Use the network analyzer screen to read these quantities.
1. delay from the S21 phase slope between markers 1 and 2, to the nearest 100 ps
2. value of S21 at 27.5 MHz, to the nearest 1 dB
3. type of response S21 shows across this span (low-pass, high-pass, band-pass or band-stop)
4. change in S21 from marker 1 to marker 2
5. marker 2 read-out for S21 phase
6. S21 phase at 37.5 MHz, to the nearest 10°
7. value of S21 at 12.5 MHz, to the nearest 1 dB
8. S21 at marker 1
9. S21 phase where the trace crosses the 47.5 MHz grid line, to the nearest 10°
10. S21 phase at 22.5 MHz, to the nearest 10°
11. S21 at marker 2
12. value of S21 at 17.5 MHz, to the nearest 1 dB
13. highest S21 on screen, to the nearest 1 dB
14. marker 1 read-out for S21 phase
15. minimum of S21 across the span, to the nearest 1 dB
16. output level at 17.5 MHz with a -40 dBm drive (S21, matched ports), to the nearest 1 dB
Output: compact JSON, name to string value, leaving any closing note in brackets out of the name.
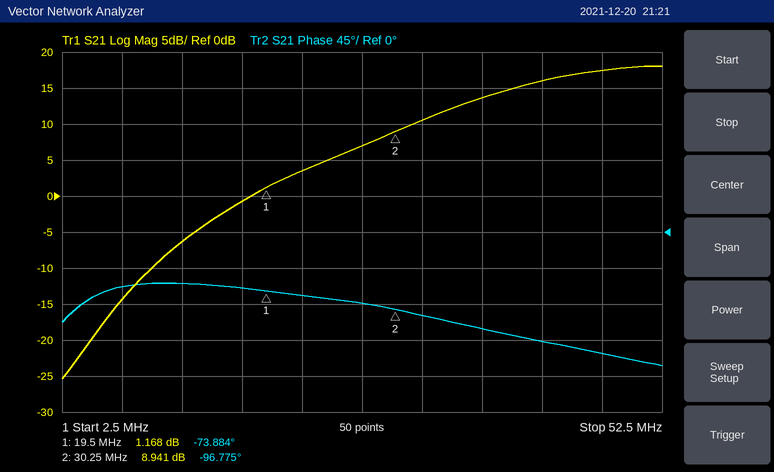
{"delay from the S21 phase slope between markers 1 and 2, to the nearest 100 ps": "5.9 ns", "value of S21 at 27.5 MHz, to the nearest 1 dB": "7 dB", "type of response S21 shows across this span": "high-pass", "change in S21 from marker 1 to marker 2": "7.773 dB", "marker 2 read-out for S21 phase": "-96.775°", "S21 phase at 37.5 MHz, to the nearest 10°": "-120°", "value of S21 at 12.5 MHz, to the nearest 1 dB": "-6 dB", "S21 at marker 1": "1.168 dB", "S21 phase where the trace crosses the 47.5 MHz grid line, to the nearest 10°": "-150°", "S21 phase at 22.5 MHz, to the nearest 10°": "-80°", "S21 at marker 2": "8.941 dB", "value of S21 at 17.5 MHz, to the nearest 1 dB": "-1 dB", "highest S21 on screen, to the nearest 1 dB": "18 dB", "marker 1 read-out for S21 phase": "-73.884°", "minimum of S21 across the span, to the nearest 1 dB": "-25 dB", "output level at 17.5 MHz with a -40 dBm drive (S21, matched ports), to the nearest 1 dB": "-41 dBm"}
